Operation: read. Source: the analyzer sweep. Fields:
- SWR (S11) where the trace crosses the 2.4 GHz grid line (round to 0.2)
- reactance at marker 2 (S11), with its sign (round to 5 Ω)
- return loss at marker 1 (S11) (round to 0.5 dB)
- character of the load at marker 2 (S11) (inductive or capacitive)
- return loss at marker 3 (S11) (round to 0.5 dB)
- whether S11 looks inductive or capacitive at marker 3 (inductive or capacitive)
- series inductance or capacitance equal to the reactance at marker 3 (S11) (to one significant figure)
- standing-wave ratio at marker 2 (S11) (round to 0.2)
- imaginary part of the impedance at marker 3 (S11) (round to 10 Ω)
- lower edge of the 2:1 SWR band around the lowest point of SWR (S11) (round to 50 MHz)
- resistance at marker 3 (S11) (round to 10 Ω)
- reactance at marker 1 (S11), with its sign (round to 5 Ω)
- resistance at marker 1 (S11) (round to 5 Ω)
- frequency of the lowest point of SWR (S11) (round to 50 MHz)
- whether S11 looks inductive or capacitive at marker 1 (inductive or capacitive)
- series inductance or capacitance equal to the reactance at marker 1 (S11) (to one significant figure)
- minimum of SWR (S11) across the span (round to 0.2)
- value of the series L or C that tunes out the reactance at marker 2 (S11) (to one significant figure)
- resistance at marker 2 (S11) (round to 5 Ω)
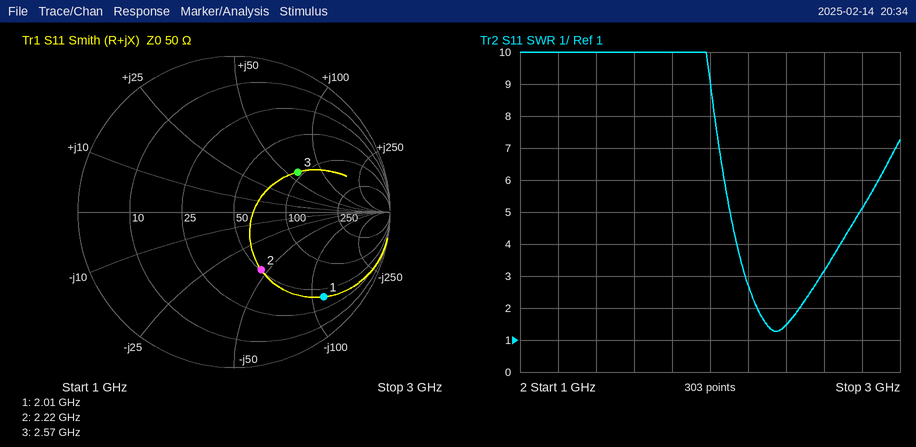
1.4
-45 Ω
2.0 dB
capacitive
6.5 dB
inductive
4 nH
2.4
+60 Ω
2.25 GHz
90 Ω
-115 Ω
40 Ω
2.35 GHz
capacitive
700 fF
1.2
3 nH
50 Ω
